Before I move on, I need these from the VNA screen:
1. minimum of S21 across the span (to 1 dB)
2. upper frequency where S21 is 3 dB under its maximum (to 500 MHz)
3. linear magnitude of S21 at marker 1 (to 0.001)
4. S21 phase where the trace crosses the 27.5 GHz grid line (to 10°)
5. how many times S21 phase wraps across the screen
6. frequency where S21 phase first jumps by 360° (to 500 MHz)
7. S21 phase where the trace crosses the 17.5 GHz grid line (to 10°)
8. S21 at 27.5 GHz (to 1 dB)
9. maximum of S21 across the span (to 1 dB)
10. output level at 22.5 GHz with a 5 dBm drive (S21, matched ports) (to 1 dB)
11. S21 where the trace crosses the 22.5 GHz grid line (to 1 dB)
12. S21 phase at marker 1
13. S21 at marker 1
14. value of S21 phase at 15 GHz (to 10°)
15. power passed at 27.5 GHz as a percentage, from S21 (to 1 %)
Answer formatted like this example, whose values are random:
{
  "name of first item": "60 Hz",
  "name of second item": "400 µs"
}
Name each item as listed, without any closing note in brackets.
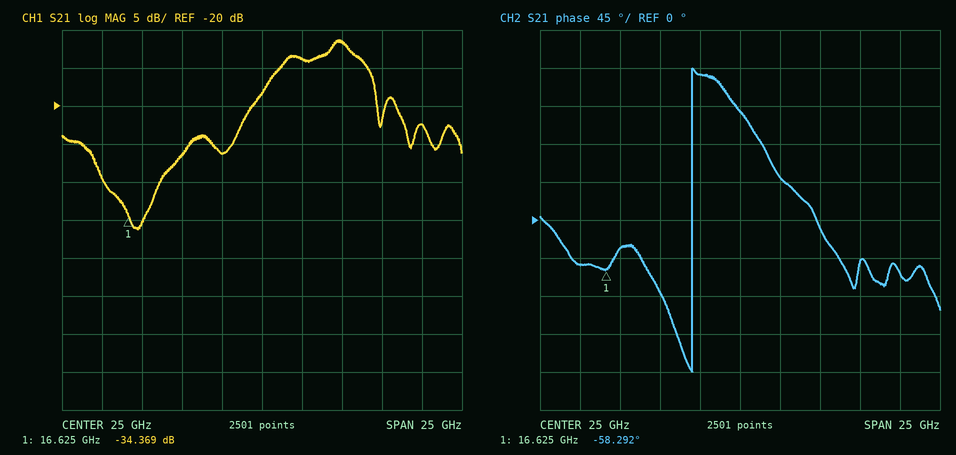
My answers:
{
  "minimum of S21 across the span": "-36 dB",
  "upper frequency where S21 is 3 dB under its maximum": "31.5 GHz",
  "linear magnitude of S21 at marker 1": "0.019",
  "S21 phase where the trace crosses the 27.5 GHz grid line": "50°",
  "how many times S21 phase wraps across the screen": "1",
  "frequency where S21 phase first jumps by 360°": "22.0 GHz",
  "S21 phase where the trace crosses the 17.5 GHz grid line": "-30°",
  "S21 at 27.5 GHz": "-14 dB",
  "maximum of S21 across the span": "-11 dB",
  "output level at 22.5 GHz with a 5 dBm drive (S21, matched ports)": "-21 dBm",
  "S21 where the trace crosses the 22.5 GHz grid line": "-26 dB",
  "S21 phase at marker 1": "-58.292°",
  "S21 at marker 1": "-34.369 dB",
  "value of S21 phase at 15 GHz": "-50°",
  "power passed at 27.5 GHz as a percentage, from S21": "4 %"
}
